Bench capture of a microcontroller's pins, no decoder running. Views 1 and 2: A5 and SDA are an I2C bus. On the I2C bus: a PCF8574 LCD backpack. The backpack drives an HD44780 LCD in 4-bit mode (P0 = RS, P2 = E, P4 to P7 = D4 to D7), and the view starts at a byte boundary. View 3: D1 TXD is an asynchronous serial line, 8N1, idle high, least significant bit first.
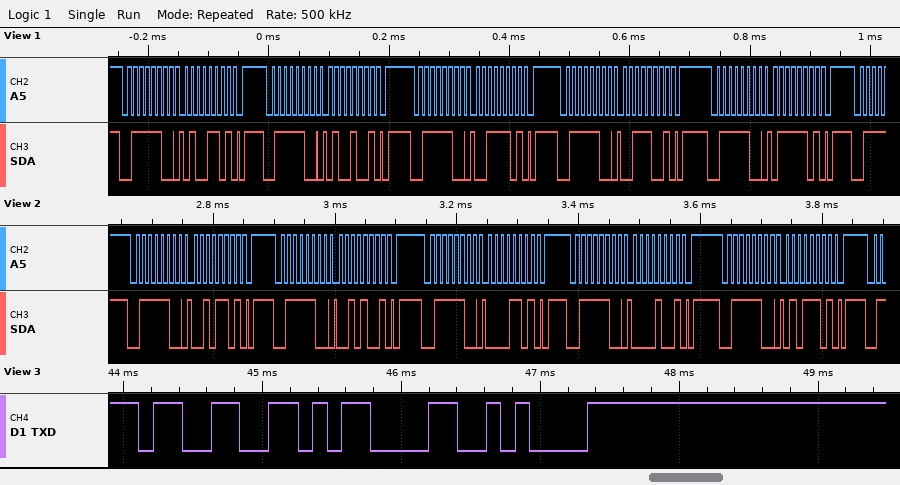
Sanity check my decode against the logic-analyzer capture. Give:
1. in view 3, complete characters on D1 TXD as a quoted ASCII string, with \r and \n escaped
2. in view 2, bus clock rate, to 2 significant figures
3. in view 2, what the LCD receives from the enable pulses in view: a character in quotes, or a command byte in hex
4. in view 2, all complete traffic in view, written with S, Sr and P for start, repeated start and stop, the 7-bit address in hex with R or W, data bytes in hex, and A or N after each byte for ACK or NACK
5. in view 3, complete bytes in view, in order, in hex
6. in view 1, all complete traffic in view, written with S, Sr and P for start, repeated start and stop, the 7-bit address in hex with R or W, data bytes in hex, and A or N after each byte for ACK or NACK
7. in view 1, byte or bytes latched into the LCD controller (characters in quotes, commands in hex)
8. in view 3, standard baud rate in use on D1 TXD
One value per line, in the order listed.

"3\r\n"
100 kHz
' '
S 3EW A 2D A P S 3EW A 29 A P S 3EW A 0D A P S 3EW A 09 A P S 3EW A 5D A P
0x33 0x0D 0x0A
S 3EW A 4D A P S 3EW A 49 A P S 3EW A 3D A P S 3EW A 39 A P S 3EW A 7D A P
'C'
9600 baud
